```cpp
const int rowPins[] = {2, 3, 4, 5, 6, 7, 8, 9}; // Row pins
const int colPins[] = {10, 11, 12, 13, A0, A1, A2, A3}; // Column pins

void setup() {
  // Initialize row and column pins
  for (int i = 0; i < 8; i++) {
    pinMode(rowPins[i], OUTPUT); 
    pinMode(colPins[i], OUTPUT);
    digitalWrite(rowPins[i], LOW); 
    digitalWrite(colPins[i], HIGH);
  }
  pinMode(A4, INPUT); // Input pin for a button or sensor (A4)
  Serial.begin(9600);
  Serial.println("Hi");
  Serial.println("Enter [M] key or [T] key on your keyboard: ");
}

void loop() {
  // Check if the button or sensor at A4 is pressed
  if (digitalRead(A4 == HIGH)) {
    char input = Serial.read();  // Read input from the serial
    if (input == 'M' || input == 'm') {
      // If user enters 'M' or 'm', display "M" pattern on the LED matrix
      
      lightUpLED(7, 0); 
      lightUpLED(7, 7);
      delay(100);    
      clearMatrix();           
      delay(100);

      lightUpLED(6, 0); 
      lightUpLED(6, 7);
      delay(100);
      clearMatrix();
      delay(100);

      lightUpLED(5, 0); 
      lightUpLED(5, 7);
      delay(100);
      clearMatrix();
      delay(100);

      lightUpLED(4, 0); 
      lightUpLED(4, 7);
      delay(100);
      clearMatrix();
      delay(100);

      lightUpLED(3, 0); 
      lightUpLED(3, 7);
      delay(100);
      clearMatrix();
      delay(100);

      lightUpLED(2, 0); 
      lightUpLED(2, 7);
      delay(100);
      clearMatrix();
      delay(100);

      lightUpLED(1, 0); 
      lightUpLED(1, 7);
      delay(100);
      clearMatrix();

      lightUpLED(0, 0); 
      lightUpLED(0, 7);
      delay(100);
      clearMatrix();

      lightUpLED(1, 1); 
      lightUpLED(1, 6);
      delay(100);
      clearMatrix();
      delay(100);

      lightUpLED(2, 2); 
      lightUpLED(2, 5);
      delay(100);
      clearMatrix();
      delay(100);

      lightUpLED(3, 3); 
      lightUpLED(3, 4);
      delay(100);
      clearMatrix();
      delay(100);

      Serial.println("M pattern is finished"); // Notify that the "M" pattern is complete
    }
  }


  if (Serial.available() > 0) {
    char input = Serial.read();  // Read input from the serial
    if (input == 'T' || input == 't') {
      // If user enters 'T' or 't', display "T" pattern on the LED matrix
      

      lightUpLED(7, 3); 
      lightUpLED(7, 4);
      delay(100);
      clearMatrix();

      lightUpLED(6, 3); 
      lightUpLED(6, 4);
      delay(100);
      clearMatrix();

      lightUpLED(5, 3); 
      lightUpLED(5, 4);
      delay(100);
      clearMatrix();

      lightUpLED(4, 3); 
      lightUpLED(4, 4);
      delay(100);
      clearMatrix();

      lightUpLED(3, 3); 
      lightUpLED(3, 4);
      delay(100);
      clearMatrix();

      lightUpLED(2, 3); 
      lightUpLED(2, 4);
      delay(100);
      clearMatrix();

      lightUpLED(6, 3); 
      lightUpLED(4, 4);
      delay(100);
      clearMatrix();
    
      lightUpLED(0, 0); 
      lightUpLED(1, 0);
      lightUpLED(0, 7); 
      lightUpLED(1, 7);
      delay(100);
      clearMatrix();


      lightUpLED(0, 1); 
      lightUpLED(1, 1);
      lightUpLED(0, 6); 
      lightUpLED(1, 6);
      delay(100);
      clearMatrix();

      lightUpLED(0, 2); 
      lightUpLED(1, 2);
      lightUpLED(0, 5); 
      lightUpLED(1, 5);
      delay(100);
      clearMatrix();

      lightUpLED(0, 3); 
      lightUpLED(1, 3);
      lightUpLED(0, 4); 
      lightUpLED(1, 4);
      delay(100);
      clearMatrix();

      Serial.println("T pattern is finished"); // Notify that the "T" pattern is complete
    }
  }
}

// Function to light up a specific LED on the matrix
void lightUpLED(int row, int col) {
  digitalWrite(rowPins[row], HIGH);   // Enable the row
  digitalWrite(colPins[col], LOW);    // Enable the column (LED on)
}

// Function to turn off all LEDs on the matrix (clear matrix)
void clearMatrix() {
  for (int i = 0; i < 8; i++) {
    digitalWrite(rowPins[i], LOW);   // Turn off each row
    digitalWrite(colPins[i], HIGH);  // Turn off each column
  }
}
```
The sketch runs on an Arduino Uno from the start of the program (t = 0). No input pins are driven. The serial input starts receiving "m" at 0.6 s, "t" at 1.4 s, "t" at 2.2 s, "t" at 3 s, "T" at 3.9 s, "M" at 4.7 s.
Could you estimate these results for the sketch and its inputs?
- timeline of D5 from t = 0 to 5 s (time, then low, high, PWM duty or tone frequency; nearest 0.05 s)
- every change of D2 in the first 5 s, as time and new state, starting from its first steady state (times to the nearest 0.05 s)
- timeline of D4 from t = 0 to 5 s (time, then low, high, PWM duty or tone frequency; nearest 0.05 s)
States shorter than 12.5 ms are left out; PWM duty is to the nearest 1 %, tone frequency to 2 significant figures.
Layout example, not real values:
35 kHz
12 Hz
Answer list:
0 s low; 1.8 s high; 1.9 s low; 2.9 s high; 3 s low; 4 s high; 4.1 s low
0 s low; 2.1 s high; 2.5 s low; 3.2 s high; 3.6 s low; 4.3 s high; 4.7 s low
0 s low; 1.9 s high; 2 s low; 3 s high; 3.1 s low; 4.1 s high; 4.2 s low
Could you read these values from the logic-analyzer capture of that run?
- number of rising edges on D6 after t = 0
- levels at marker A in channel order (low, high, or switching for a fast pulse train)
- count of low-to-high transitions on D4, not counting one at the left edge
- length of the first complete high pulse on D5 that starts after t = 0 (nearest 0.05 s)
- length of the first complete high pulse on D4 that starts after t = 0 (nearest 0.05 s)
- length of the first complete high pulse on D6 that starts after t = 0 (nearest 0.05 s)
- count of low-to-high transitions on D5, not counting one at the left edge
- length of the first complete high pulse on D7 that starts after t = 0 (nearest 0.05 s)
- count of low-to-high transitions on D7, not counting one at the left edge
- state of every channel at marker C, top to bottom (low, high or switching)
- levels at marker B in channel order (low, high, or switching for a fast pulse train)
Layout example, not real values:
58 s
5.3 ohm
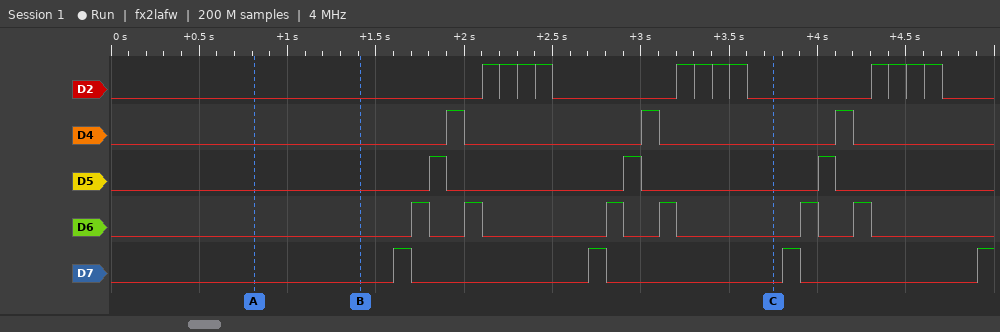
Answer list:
6
D2 low, D4 low, D5 low, D6 low, D7 low
3
0.10 s
0.10 s
0.10 s
3
0.10 s
4
D2 low, D4 low, D5 low, D6 low, D7 low
D2 low, D4 low, D5 low, D6 low, D7 low
